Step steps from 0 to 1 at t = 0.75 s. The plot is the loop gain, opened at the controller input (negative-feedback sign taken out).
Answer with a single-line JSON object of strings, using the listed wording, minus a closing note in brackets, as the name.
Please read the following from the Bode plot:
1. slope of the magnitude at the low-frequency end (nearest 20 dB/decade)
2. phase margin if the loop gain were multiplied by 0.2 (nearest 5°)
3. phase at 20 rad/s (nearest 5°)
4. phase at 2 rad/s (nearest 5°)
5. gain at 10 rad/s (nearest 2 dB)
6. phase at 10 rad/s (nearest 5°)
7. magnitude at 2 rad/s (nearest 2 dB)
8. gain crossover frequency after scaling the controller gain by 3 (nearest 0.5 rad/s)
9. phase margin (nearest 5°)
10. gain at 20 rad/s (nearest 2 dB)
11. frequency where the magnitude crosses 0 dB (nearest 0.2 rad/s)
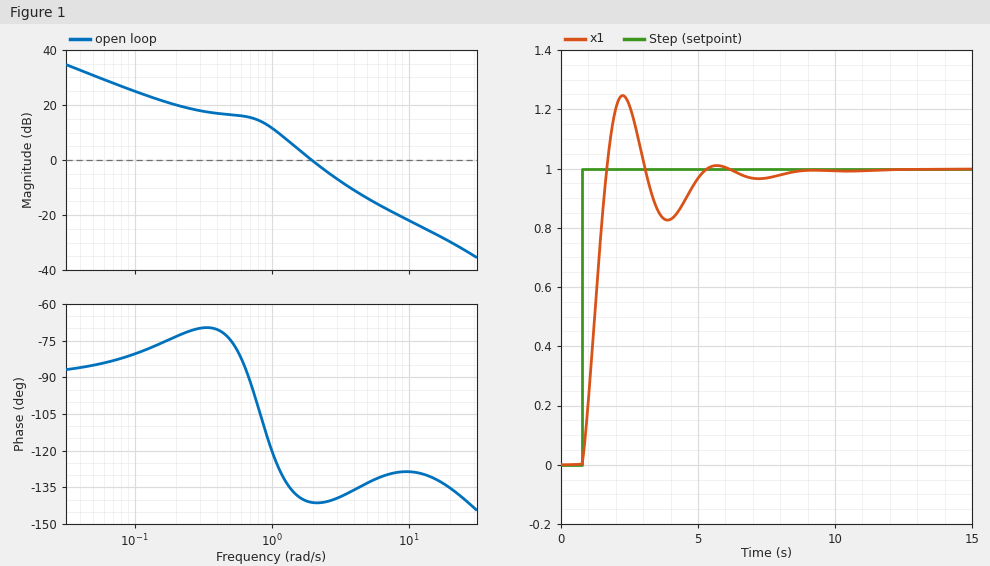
{"slope of the magnitude at the low-frequency end": "-20 dB/decade", "phase margin if the loop gain were multiplied by 0.2": "75°", "phase at 20 rad/s": "-135°", "phase at 2 rad/s": "-140°", "gain at 10 rad/s": "-22 dB", "phase at 10 rad/s": "-130°", "magnitude at 2 rad/s": "0 dB", "gain crossover frequency after scaling the controller gain by 3": "3.5 rad/s", "phase margin": "40°", "gain at 20 rad/s": "-30 dB", "frequency where the magnitude crosses 0 dB": "2.0 rad/s"}
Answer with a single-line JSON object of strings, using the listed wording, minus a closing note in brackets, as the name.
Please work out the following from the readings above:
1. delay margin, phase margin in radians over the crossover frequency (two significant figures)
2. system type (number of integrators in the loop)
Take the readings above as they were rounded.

{"delay margin, phase margin in radians over the crossover frequency": "0.35 s", "system type": "1"}
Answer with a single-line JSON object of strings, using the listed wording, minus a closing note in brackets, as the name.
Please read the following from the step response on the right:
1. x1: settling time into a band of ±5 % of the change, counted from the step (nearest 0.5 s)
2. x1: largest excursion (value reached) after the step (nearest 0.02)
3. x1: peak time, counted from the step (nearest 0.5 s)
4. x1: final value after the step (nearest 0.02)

{"x1: settling time into a band of ±5 % of the change, counted from the step": "4.0 s", "x1: largest excursion (value reached) after the step": "1.24", "x1: peak time, counted from the step": "1.5 s", "x1: final value after the step": "1.00"}
